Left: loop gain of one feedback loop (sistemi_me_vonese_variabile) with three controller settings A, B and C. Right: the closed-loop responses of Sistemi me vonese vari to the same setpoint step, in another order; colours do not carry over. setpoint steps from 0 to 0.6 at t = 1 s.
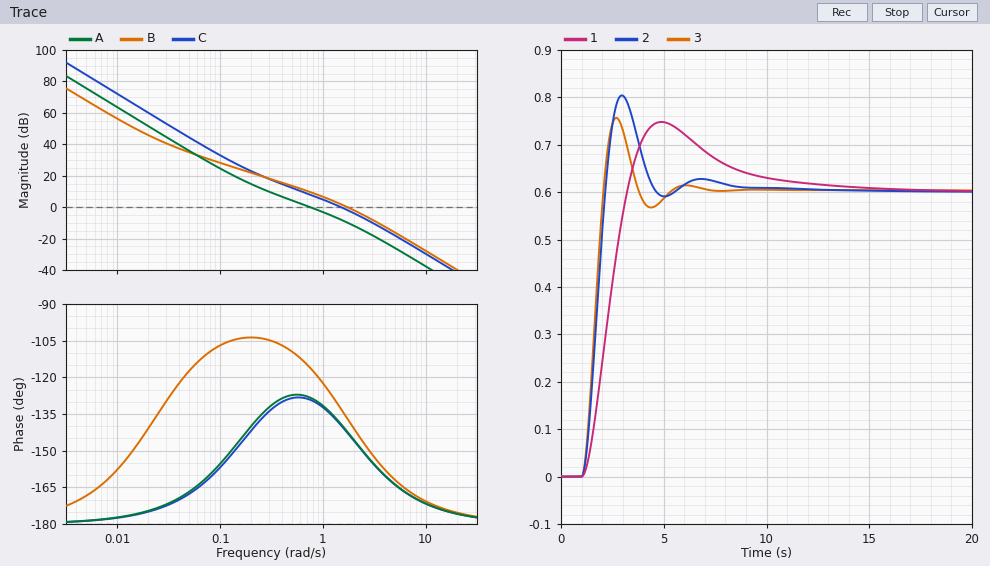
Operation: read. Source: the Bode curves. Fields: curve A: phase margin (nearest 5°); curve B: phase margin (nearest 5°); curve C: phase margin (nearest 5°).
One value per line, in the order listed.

50°
45°
40°
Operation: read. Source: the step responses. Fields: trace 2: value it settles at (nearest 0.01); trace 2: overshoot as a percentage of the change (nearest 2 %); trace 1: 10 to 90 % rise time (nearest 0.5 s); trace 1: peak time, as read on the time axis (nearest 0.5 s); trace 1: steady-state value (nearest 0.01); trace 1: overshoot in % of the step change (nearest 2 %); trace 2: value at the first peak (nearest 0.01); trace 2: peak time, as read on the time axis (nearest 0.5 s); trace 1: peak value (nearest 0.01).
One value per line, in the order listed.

0.60
34 %
1.5 s
5.0 s
0.60
24 %
0.80
3.0 s
0.75
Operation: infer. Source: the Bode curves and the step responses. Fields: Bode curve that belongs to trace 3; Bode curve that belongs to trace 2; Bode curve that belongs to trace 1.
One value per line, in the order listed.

B
C
A
